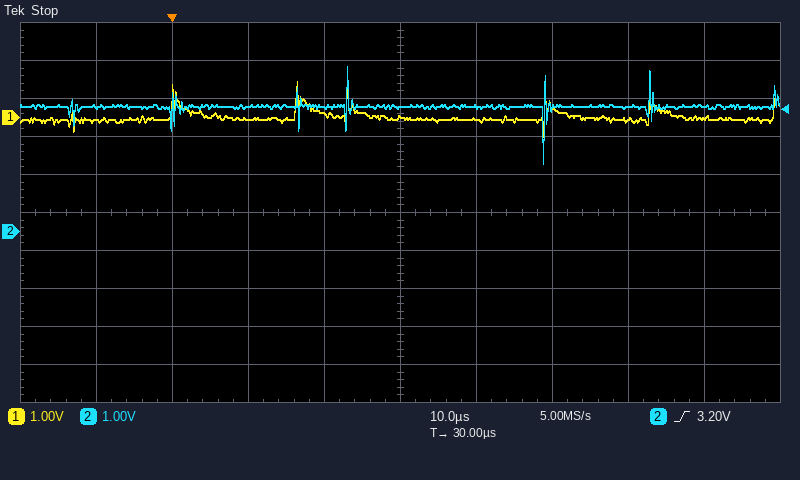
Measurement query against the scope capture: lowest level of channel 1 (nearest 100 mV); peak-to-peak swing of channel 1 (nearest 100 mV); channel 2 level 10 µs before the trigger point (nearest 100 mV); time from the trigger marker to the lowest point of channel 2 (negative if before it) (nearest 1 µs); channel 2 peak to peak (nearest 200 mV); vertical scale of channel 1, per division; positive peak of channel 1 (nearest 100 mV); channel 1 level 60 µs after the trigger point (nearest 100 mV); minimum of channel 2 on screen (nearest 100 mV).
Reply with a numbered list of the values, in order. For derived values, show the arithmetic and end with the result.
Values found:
1. -500 mV
2. 900 mV − (-500 mV) = 1.4 V
3. 3.3 V
4. +49 µs
5. 2.6 V
6. 1 V
7. 900 mV
8. -100 mV
9. 1.8 V
